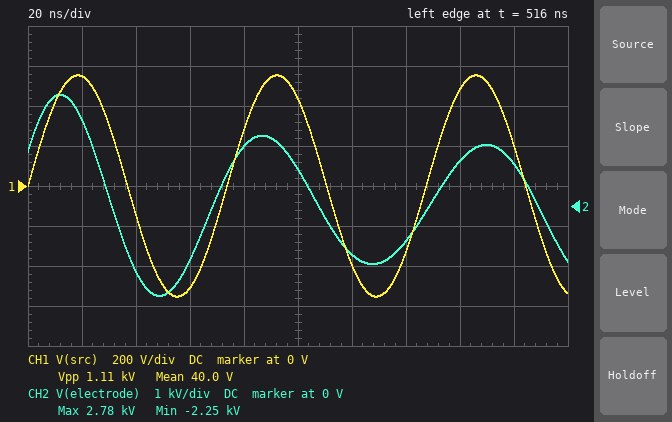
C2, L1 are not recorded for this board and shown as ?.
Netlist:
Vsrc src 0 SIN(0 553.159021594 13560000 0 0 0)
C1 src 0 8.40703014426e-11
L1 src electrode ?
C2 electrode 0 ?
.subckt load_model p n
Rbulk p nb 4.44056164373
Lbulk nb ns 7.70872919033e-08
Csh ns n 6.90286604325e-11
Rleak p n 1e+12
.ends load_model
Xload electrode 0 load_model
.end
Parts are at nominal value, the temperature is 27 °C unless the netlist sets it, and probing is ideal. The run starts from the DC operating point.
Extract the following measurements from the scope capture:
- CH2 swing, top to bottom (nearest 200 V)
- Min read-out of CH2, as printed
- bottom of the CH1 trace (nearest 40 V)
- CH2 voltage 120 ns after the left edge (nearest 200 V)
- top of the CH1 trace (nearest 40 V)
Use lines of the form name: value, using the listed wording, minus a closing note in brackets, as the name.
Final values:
CH2 swing, top to bottom: 5.0 kV
Min read-out of CH2, as printed: -2.25 kV
bottom of the CH1 trace: -560 V
CH2 voltage 120 ns after the left edge: -1.2 kV
top of the CH1 trace: 560 V
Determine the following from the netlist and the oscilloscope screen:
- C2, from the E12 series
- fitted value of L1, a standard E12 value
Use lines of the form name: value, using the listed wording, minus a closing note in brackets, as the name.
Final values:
C2, from the E12 series: 39 pF
fitted value of L1, a standard E12 value: 1 µH
